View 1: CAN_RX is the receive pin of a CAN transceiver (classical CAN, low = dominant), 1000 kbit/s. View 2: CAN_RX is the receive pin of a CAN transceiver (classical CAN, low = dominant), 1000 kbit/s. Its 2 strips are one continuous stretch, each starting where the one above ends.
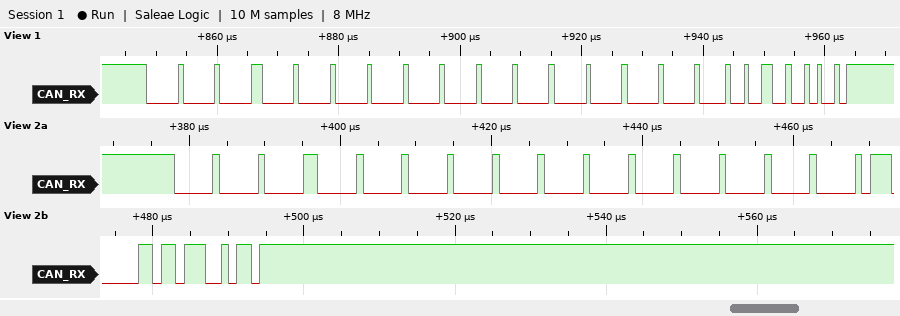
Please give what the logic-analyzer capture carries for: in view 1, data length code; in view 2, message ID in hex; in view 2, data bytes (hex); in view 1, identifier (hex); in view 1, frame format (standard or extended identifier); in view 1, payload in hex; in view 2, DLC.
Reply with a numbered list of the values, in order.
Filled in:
1. 8
2. 0x000
3. 00 00 00 00 00 00 00 38
4. 0x000
5. standard
6. 00 00 00 00 00 00 00 04
7. 8
